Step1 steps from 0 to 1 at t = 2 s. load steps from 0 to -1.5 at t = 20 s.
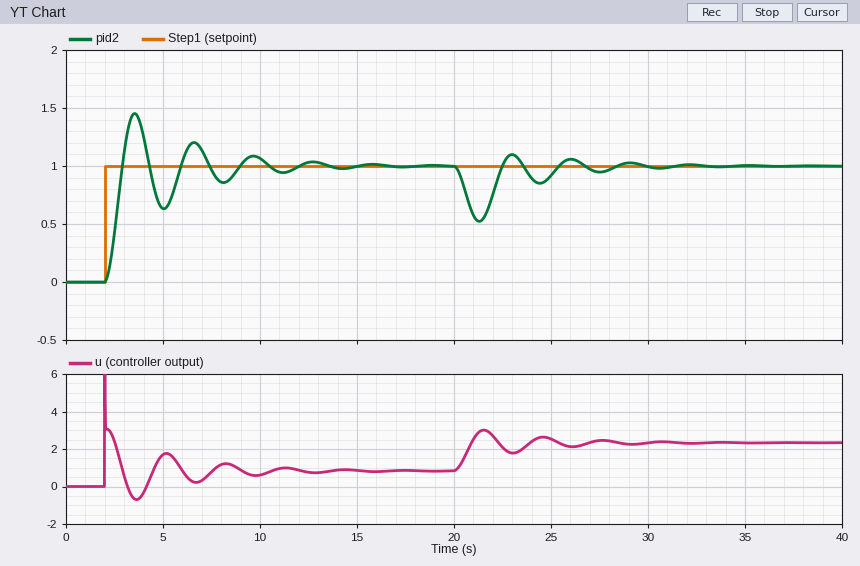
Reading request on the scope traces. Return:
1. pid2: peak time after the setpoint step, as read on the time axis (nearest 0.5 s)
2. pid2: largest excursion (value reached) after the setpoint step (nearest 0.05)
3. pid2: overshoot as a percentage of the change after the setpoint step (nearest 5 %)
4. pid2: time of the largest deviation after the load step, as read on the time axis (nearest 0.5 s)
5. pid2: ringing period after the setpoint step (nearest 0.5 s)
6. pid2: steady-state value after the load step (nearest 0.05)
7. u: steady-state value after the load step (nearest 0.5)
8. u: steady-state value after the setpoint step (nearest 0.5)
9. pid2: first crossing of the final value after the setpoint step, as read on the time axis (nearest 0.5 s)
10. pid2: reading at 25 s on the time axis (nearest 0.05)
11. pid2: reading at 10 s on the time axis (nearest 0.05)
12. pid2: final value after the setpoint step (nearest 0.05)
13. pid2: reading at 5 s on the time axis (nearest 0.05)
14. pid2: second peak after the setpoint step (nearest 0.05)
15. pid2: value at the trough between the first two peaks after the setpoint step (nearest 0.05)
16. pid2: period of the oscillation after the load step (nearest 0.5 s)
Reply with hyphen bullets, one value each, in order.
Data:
- 3.5 s
- 1.45
- 45 %
- 21.5 s
- 3.0 s
- 1.00
- 2.5
- 1.0
- 3.0 s
- 0.90
- 1.05
- 1.00
- 0.65
- 1.20
- 0.65
- 3.0 s
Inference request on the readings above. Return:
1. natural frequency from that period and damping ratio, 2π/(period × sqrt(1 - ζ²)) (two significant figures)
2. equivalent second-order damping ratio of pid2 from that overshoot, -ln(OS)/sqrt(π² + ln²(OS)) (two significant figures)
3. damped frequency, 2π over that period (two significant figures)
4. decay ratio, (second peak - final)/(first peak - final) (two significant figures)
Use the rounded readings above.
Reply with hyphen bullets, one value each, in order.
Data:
- 2.2 rad/s
- 0.25
- 2.1 rad/s
- 0.44
